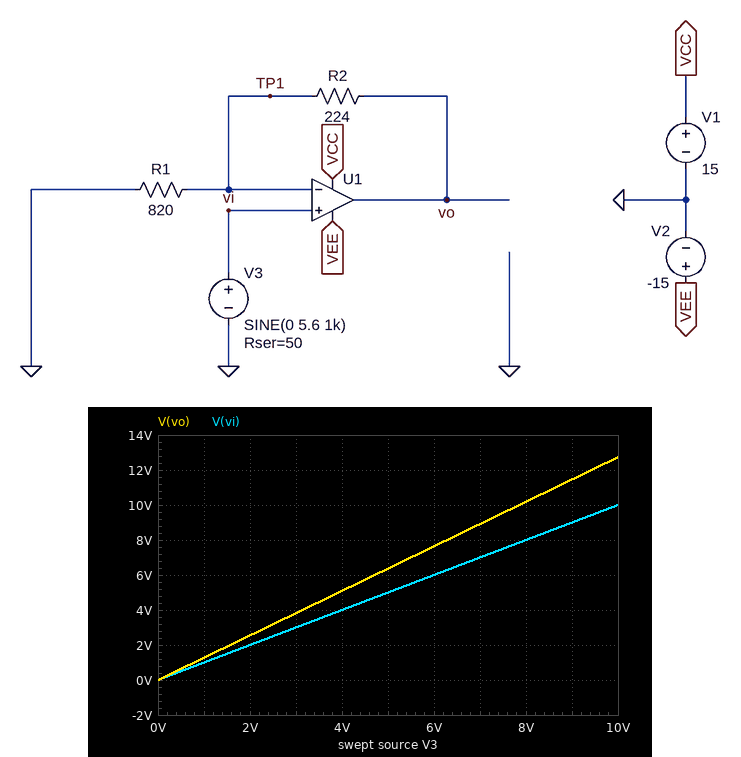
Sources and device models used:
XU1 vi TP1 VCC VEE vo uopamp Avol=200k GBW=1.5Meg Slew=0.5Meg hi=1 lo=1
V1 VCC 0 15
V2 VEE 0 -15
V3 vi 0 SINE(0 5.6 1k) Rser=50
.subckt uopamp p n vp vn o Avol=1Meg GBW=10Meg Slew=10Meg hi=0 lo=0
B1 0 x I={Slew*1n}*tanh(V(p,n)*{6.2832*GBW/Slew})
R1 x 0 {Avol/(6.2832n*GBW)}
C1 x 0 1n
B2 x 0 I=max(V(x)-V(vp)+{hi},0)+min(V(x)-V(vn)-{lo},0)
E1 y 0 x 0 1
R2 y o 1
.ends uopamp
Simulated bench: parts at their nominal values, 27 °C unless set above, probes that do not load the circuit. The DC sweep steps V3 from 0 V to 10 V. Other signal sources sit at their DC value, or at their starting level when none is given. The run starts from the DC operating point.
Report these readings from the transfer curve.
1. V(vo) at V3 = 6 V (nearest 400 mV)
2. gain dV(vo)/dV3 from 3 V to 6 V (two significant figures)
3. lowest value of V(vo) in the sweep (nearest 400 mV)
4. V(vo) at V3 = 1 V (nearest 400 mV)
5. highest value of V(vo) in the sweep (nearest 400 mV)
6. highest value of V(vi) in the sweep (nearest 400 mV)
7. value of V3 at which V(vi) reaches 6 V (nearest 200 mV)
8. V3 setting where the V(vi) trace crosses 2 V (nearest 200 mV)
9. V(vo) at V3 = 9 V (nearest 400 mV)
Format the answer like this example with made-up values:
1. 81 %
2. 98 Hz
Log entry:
1. 7.6 V
2. 1.3 V/V
3. 0 V
4. 1.2 V
5. 12.8 V
6. 10.0 V
7. 6.0 V
8. 2.0 V
9. 11.6 V
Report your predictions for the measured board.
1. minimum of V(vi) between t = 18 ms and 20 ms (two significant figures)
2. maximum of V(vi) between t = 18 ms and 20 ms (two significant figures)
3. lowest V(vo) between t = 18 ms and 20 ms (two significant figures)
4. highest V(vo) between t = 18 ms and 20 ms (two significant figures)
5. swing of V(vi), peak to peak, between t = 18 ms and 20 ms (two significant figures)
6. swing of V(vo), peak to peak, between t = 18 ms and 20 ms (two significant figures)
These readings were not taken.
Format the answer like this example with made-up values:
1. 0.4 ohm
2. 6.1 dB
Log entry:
1. -5.6 V
2. 5.6 V
3. -7.1 V
4. 7.1 V
5. 11 V
6. 14 V
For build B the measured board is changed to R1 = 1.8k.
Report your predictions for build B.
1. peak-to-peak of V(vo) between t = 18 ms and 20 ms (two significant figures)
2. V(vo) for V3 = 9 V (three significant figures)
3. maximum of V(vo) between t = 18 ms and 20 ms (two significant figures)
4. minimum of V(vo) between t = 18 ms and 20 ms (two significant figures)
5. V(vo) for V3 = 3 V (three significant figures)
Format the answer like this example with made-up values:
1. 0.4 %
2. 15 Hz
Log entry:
1. 13 V
2. 10.1 V
3. 6.3 V
4. -6.3 V
5. 3.37 V
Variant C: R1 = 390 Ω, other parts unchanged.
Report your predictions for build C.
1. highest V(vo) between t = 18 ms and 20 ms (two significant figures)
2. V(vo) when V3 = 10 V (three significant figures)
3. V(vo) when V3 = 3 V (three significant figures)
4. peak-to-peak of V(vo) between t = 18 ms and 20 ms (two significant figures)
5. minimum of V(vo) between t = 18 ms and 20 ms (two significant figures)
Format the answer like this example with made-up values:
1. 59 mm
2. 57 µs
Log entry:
1. 8.8 V
2. 14.0 V
3. 4.72 V
4. 18 V
5. -8.8 V
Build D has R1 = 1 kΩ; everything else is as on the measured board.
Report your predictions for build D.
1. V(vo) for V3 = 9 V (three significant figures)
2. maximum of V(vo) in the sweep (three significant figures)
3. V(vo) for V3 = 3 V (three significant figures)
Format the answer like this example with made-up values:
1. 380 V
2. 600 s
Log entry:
1. 11.0 V
2. 12.2 V
3. 3.67 V
